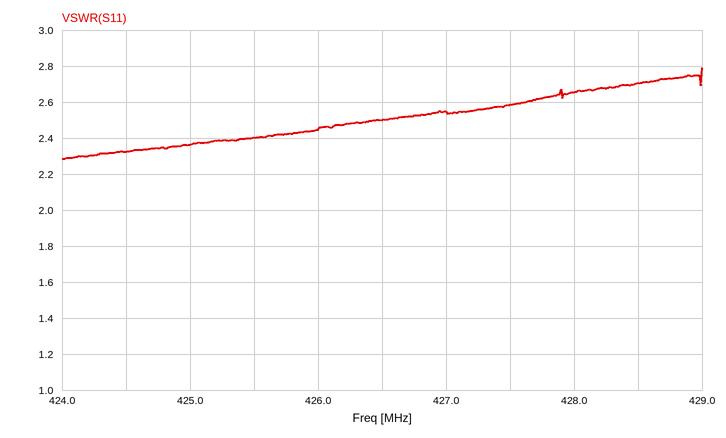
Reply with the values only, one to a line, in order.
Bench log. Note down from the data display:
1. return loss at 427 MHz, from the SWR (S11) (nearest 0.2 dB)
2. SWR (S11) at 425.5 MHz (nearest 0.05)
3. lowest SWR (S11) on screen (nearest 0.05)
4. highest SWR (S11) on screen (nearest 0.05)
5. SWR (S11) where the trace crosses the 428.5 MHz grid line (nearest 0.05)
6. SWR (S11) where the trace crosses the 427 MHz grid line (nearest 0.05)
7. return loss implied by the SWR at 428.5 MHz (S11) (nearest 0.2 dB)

7.2 dB
2.40
2.30
2.80
2.70
2.55
6.8 dB
